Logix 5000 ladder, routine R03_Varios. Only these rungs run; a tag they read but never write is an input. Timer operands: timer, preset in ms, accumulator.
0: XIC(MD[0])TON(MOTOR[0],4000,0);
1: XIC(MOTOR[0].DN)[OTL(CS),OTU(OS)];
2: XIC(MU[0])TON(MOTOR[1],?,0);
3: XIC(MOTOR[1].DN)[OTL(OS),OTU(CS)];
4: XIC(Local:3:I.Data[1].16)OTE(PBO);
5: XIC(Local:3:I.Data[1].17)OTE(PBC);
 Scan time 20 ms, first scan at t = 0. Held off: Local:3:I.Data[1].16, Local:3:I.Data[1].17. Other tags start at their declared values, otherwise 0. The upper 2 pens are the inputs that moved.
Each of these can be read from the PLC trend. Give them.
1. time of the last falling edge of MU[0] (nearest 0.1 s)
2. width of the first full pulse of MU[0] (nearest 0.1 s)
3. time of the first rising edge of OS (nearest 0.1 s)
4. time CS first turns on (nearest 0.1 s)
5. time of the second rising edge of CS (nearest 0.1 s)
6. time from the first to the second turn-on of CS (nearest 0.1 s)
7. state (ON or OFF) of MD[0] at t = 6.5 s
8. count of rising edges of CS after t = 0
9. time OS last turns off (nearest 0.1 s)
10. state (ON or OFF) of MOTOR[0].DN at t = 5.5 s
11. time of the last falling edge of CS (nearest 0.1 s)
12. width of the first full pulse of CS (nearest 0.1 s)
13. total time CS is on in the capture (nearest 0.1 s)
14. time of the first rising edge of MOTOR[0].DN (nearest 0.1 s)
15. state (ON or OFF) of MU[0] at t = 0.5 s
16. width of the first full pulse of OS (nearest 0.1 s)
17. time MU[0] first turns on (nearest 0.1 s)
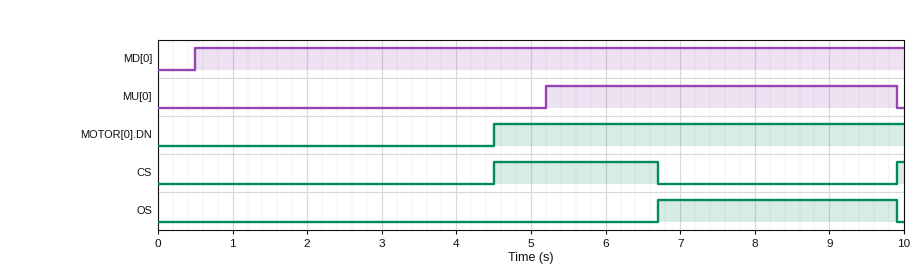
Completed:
9.9 s
4.7 s
6.7 s
4.5 s
9.9 s
5.4 s
ON
2
9.9 s
ON
6.7 s
2.2 s
2.3 s
4.5 s
OFF
3.2 s
5.2 s
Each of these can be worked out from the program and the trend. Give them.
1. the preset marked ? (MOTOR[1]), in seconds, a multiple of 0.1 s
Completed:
1.5 s
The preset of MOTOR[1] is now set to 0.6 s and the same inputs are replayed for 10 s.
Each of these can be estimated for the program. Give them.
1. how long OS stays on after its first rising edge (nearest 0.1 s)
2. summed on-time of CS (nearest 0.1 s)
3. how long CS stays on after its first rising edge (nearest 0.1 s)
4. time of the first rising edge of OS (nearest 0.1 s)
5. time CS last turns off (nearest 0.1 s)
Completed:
4.1 s
1.4 s
1.3 s
5.8 s
5.8 s
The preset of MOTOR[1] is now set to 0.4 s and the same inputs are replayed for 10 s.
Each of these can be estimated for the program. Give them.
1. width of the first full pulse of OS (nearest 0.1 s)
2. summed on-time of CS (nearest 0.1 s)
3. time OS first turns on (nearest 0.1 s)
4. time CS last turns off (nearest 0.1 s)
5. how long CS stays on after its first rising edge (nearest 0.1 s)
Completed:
4.3 s
1.2 s
5.6 s
5.6 s
1.1 s
